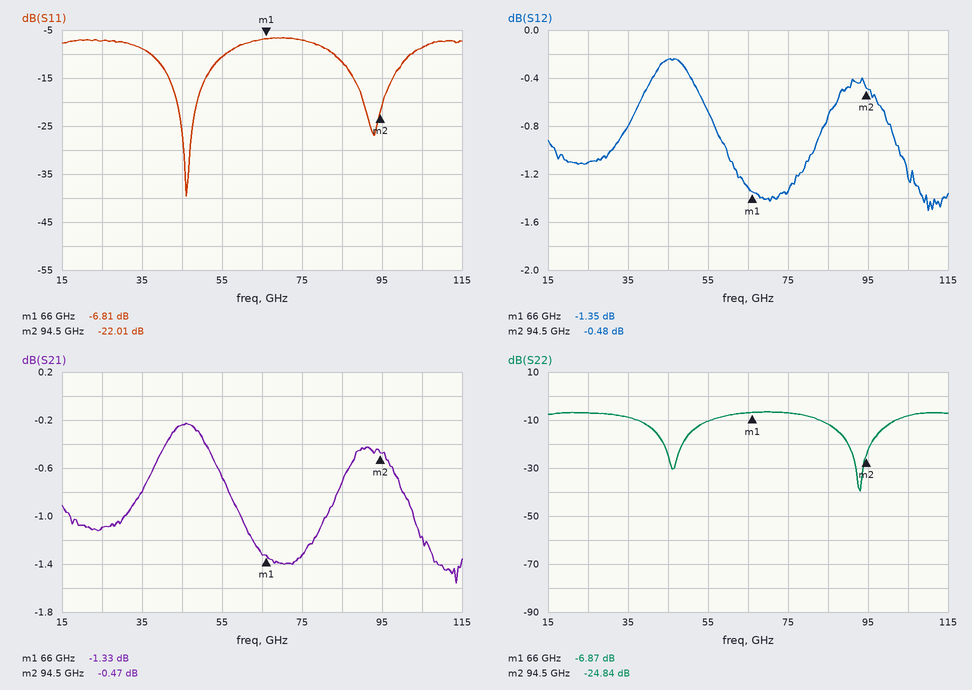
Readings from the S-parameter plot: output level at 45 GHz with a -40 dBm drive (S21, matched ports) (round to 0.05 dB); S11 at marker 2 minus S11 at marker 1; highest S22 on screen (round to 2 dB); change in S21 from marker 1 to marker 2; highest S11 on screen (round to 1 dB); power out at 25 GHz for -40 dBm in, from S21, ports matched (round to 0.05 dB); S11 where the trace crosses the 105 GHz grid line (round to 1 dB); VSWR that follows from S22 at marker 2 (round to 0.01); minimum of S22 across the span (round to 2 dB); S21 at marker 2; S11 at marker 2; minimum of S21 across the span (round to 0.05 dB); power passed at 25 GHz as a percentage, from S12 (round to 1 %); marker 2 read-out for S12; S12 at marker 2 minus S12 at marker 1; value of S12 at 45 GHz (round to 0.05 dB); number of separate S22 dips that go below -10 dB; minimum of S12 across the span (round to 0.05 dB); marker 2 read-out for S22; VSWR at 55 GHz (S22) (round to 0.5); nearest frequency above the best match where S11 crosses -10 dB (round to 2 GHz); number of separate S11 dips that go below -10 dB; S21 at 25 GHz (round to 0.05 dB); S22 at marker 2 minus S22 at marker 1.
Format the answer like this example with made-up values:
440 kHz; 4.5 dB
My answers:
-40.25 dBm; -15.20 dB; -6 dB; 0.86 dB; -7 dB; -41.10 dBm; -9 dB; 1.12; -40 dB; -0.47 dB; -22.01 dB; -1.55 dB; 78 %; -0.48 dB; 0.87 dB; -0.25 dB; 2; -1.50 dB; -24.84 dB; 2.0; 56 GHz; 2; -1.10 dB; -17.97 dB
